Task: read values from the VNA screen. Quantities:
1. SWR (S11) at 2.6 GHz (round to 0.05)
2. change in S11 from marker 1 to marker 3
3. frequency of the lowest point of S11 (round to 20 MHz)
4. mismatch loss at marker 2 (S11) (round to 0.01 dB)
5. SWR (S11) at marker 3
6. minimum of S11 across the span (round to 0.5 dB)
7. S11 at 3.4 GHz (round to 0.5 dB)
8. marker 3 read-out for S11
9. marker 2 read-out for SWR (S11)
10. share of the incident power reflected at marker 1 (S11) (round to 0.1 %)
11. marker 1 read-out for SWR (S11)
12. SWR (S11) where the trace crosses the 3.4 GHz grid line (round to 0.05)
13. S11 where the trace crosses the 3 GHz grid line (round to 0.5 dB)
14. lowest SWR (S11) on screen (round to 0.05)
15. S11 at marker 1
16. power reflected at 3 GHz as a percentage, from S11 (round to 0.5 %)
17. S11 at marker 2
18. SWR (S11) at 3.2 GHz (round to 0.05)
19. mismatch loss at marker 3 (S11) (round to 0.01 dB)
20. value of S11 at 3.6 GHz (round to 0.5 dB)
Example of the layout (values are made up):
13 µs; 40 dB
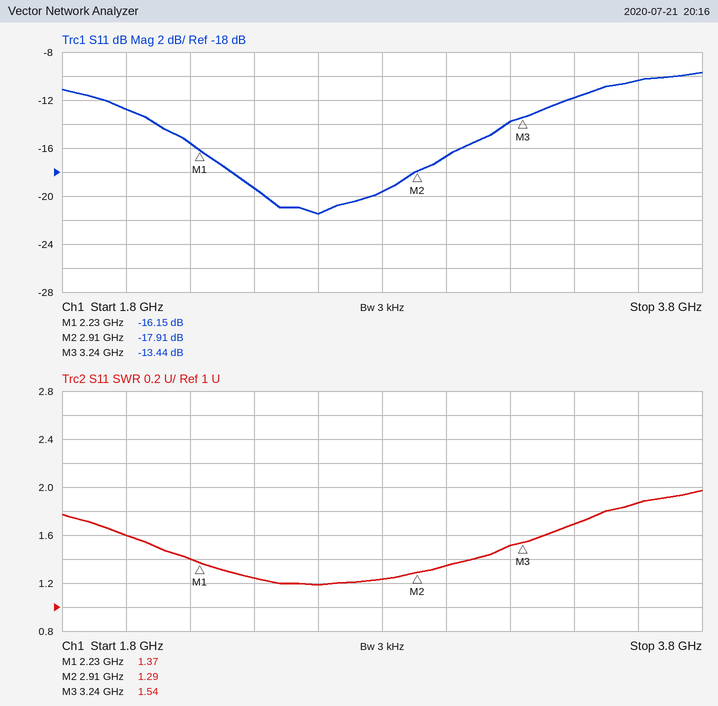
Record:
1.20; 2.71 dB; 2.60 GHz; 0.07 dB; 1.54; -21.5 dB; -12.0 dB; -13.44 dB; 1.29; 2.4 %; 1.37; 1.70; -16.5 dB; 1.20; -16.15 dB; 2.0 %; -17.91 dB; 1.50; 0.20 dB; -10.5 dB
